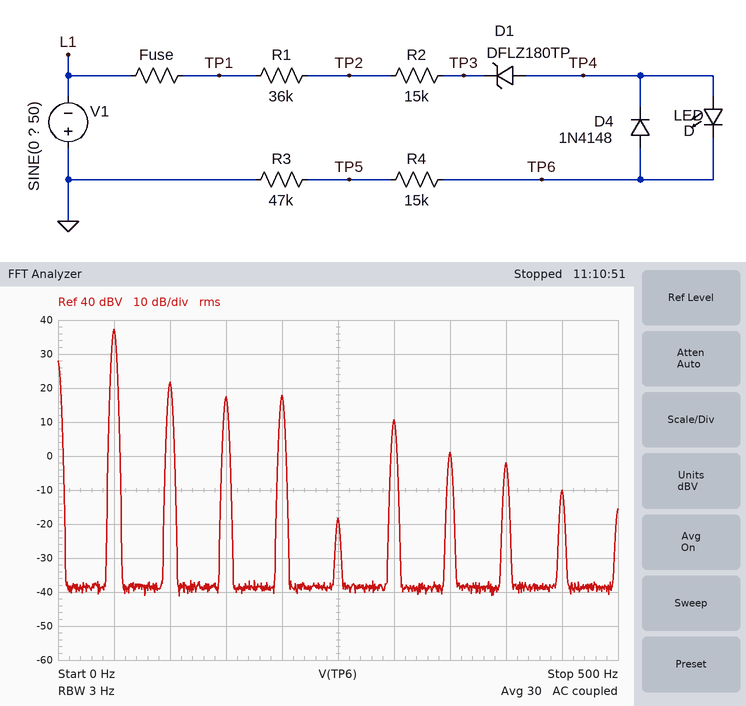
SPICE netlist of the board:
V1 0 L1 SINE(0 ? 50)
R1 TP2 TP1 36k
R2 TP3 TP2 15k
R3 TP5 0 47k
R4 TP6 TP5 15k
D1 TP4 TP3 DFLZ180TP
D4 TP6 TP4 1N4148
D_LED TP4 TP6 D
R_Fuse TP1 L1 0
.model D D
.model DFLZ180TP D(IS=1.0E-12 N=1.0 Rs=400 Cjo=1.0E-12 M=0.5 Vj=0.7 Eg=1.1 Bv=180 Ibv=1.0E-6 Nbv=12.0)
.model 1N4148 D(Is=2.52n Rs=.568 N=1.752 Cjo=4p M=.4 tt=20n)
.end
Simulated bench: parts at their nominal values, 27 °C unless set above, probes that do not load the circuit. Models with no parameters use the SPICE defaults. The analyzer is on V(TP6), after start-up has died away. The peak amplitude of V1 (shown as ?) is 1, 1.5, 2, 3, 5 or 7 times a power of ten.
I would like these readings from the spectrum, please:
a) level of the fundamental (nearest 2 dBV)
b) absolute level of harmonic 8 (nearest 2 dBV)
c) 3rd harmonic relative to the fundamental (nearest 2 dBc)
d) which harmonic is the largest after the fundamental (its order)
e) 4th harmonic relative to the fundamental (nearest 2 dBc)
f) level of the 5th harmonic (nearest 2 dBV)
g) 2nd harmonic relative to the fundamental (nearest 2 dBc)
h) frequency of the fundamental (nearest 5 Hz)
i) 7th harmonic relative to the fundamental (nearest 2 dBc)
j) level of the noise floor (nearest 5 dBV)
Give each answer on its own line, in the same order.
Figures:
38 dBV
-2 dBV
-20 dBc
2
-20 dBc
-18 dBV
-16 dBc
50 Hz
-36 dBc
-40 dBV
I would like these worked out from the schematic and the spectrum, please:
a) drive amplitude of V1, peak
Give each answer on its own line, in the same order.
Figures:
300 V
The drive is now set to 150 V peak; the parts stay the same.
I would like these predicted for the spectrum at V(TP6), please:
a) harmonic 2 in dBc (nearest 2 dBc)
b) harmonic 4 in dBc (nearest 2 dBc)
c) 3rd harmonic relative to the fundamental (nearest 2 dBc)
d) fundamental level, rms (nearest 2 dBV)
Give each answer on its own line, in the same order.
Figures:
-8 dBc
-22 dBc
-50 dBc
30 dBV
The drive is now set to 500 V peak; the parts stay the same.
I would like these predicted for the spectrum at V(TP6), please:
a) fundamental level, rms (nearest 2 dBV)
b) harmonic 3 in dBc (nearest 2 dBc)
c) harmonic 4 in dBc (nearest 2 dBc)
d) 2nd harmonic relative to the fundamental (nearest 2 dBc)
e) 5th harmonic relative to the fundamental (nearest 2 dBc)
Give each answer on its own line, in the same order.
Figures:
44 dBV
-22 dBc
-26 dBc
-26 dBc
-30 dBc
